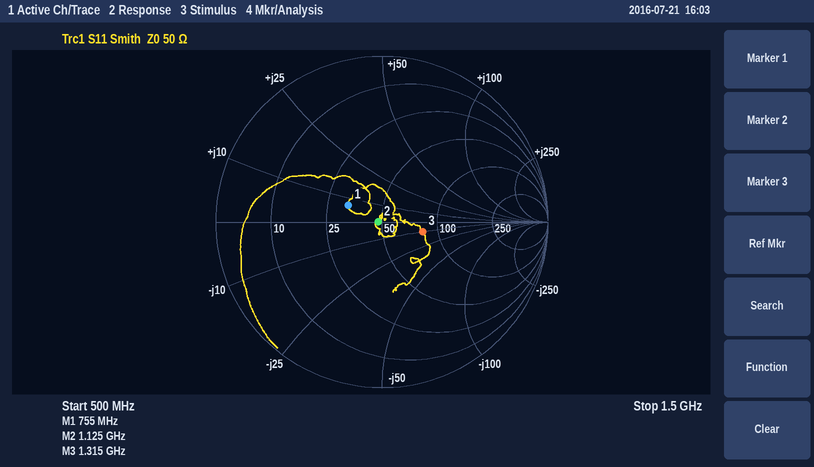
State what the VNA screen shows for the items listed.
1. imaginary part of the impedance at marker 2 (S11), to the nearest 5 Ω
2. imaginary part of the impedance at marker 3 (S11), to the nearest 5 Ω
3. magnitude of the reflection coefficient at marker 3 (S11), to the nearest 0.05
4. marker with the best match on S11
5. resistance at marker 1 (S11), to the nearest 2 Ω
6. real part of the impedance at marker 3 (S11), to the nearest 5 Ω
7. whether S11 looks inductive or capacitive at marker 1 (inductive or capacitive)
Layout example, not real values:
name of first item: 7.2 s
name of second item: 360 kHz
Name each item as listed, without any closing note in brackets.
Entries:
imaginary part of the impedance at marker 2 (S11), to the nearest 5 Ω: 0 Ω
imaginary part of the impedance at marker 3 (S11), to the nearest 5 Ω: -10 Ω
magnitude of the reflection coefficient at marker 3 (S11), to the nearest 0.05: 0.25
marker with the best match on S11: marker 2
resistance at marker 1 (S11), to the nearest 2 Ω: 32 Ω
real part of the impedance at marker 3 (S11), to the nearest 5 Ω: 80 Ω
whether S11 looks inductive or capacitive at marker 1: inductive
